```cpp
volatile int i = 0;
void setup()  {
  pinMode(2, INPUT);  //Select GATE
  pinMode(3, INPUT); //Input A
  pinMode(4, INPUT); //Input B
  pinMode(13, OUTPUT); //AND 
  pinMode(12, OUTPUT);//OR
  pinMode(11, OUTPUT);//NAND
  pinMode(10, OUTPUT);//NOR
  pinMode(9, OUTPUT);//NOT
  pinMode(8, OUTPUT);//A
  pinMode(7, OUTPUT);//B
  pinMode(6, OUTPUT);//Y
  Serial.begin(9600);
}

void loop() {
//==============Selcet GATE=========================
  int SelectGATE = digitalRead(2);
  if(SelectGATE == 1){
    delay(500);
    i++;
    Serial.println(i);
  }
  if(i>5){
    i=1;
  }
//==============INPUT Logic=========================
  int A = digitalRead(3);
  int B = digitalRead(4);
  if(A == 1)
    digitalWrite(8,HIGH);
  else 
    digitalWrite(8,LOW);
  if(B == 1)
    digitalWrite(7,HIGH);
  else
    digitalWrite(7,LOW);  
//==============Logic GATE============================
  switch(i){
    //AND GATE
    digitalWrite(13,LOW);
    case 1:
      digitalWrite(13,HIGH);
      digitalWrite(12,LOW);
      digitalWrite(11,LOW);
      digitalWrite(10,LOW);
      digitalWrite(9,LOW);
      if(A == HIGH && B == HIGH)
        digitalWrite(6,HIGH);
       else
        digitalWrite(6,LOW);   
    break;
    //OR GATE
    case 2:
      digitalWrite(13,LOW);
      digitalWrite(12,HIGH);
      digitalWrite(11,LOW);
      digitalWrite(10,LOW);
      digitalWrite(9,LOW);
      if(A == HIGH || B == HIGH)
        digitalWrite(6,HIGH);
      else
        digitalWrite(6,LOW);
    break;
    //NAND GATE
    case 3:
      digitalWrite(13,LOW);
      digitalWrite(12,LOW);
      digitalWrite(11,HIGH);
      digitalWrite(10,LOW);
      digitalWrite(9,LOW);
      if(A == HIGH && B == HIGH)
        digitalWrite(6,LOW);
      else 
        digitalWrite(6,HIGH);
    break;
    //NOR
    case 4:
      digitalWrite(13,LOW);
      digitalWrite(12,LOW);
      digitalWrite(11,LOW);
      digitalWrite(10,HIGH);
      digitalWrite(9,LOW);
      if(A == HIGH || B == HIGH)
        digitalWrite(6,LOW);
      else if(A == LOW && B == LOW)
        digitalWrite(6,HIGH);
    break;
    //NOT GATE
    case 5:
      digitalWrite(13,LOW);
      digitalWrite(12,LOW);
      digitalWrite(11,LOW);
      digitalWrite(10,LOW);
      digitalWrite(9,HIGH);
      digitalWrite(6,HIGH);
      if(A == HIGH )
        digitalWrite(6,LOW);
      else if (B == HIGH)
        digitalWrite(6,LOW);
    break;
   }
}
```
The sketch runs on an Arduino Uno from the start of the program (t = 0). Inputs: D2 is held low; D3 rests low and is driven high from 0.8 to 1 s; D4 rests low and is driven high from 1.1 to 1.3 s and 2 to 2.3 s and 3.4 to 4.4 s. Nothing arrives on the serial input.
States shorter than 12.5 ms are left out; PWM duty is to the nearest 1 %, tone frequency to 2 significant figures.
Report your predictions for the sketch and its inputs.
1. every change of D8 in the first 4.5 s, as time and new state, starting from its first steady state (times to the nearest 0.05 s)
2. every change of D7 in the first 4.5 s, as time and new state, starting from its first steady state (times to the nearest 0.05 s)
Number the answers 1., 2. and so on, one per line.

1. 0 s low; 0.8 s high; 1 s low
2. 0 s low; 1.1 s high; 1.3 s low; 2 s high; 2.3 s low; 3.4 s high; 4.4 s low
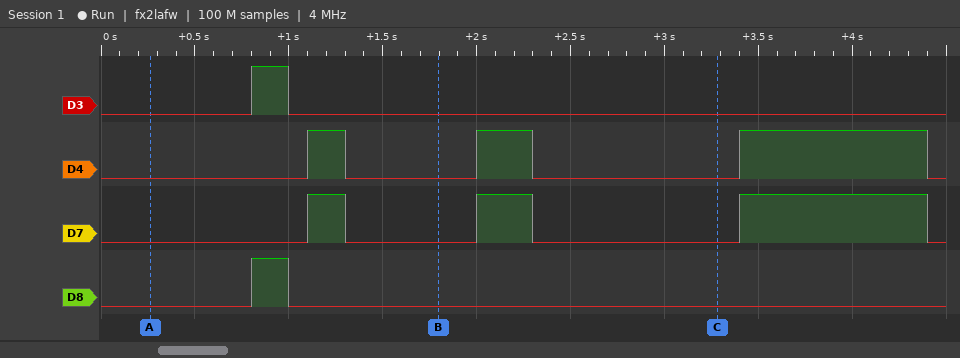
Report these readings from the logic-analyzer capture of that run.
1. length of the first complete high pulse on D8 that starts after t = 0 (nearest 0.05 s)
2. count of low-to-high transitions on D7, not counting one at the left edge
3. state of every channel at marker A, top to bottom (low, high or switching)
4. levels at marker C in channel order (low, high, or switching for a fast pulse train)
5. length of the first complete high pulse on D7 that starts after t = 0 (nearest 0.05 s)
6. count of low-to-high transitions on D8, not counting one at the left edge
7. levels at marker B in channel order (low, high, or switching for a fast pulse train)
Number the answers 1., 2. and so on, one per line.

1. 0.20 s
2. 3
3. D3 low, D4 low, D7 low, D8 low
4. D3 low, D4 low, D7 low, D8 low
5. 0.20 s
6. 1
7. D3 low, D4 low, D7 low, D8 low
